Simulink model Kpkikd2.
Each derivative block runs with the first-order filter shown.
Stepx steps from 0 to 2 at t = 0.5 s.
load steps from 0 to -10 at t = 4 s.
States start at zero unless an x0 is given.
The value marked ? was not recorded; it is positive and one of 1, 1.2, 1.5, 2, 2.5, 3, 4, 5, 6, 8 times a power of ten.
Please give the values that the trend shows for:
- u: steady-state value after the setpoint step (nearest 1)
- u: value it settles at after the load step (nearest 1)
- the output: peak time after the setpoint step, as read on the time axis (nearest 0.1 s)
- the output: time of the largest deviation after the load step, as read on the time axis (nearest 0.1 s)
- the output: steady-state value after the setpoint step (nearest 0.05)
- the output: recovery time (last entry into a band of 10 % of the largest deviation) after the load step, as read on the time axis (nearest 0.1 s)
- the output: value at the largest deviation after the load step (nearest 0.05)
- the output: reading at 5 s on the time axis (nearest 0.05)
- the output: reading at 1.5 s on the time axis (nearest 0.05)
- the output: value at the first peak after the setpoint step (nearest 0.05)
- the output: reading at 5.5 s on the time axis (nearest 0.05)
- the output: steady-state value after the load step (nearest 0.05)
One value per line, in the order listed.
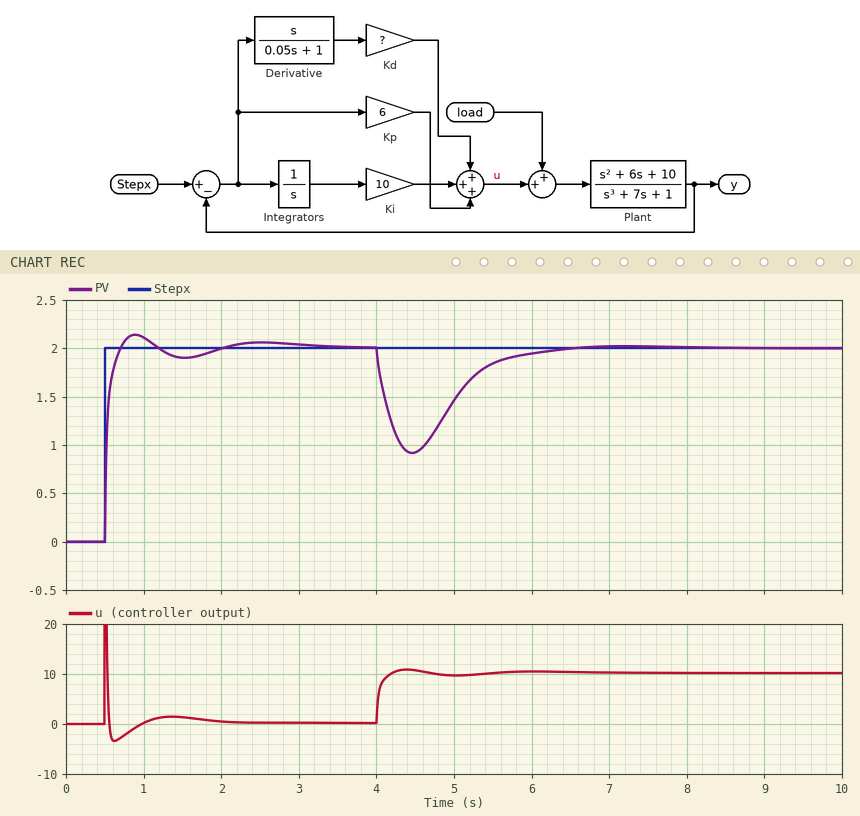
0
10
0.9 s
4.5 s
2.00
5.7 s
0.90
1.45
1.90
2.15
1.85
2.00
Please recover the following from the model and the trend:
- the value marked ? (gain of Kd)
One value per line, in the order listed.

1.5
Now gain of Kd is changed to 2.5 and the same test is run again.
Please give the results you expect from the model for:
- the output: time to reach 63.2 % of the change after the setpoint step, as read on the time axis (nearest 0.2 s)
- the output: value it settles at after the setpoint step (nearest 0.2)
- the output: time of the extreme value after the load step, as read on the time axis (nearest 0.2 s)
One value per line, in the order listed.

0.6 s
2.0
4.6 s
